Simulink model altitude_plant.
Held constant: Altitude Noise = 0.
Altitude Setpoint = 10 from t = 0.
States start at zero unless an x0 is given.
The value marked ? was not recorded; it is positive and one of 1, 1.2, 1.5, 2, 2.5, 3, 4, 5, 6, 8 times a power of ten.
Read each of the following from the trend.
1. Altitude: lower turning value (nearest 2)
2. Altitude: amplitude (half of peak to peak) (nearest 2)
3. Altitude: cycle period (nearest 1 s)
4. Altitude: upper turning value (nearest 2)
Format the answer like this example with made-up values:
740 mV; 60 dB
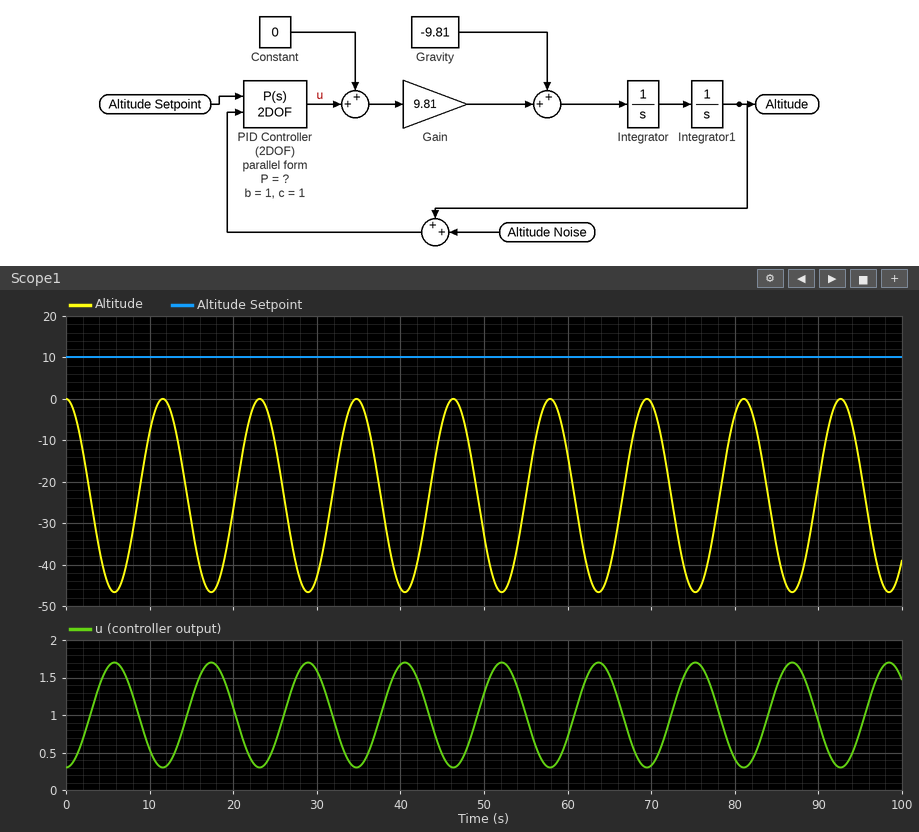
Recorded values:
-46; 24; 12 s; 0
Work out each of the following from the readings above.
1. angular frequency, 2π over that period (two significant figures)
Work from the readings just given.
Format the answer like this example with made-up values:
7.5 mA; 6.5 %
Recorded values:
0.52 rad/s
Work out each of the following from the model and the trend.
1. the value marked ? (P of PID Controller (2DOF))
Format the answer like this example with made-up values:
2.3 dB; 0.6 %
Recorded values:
0.03
